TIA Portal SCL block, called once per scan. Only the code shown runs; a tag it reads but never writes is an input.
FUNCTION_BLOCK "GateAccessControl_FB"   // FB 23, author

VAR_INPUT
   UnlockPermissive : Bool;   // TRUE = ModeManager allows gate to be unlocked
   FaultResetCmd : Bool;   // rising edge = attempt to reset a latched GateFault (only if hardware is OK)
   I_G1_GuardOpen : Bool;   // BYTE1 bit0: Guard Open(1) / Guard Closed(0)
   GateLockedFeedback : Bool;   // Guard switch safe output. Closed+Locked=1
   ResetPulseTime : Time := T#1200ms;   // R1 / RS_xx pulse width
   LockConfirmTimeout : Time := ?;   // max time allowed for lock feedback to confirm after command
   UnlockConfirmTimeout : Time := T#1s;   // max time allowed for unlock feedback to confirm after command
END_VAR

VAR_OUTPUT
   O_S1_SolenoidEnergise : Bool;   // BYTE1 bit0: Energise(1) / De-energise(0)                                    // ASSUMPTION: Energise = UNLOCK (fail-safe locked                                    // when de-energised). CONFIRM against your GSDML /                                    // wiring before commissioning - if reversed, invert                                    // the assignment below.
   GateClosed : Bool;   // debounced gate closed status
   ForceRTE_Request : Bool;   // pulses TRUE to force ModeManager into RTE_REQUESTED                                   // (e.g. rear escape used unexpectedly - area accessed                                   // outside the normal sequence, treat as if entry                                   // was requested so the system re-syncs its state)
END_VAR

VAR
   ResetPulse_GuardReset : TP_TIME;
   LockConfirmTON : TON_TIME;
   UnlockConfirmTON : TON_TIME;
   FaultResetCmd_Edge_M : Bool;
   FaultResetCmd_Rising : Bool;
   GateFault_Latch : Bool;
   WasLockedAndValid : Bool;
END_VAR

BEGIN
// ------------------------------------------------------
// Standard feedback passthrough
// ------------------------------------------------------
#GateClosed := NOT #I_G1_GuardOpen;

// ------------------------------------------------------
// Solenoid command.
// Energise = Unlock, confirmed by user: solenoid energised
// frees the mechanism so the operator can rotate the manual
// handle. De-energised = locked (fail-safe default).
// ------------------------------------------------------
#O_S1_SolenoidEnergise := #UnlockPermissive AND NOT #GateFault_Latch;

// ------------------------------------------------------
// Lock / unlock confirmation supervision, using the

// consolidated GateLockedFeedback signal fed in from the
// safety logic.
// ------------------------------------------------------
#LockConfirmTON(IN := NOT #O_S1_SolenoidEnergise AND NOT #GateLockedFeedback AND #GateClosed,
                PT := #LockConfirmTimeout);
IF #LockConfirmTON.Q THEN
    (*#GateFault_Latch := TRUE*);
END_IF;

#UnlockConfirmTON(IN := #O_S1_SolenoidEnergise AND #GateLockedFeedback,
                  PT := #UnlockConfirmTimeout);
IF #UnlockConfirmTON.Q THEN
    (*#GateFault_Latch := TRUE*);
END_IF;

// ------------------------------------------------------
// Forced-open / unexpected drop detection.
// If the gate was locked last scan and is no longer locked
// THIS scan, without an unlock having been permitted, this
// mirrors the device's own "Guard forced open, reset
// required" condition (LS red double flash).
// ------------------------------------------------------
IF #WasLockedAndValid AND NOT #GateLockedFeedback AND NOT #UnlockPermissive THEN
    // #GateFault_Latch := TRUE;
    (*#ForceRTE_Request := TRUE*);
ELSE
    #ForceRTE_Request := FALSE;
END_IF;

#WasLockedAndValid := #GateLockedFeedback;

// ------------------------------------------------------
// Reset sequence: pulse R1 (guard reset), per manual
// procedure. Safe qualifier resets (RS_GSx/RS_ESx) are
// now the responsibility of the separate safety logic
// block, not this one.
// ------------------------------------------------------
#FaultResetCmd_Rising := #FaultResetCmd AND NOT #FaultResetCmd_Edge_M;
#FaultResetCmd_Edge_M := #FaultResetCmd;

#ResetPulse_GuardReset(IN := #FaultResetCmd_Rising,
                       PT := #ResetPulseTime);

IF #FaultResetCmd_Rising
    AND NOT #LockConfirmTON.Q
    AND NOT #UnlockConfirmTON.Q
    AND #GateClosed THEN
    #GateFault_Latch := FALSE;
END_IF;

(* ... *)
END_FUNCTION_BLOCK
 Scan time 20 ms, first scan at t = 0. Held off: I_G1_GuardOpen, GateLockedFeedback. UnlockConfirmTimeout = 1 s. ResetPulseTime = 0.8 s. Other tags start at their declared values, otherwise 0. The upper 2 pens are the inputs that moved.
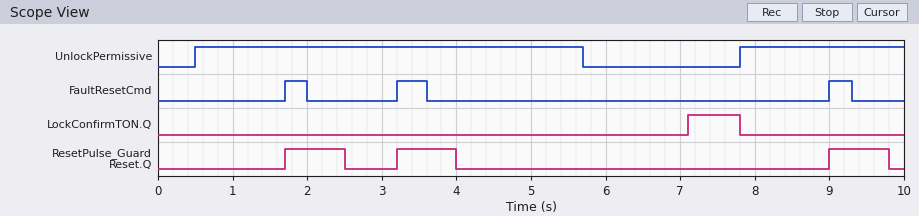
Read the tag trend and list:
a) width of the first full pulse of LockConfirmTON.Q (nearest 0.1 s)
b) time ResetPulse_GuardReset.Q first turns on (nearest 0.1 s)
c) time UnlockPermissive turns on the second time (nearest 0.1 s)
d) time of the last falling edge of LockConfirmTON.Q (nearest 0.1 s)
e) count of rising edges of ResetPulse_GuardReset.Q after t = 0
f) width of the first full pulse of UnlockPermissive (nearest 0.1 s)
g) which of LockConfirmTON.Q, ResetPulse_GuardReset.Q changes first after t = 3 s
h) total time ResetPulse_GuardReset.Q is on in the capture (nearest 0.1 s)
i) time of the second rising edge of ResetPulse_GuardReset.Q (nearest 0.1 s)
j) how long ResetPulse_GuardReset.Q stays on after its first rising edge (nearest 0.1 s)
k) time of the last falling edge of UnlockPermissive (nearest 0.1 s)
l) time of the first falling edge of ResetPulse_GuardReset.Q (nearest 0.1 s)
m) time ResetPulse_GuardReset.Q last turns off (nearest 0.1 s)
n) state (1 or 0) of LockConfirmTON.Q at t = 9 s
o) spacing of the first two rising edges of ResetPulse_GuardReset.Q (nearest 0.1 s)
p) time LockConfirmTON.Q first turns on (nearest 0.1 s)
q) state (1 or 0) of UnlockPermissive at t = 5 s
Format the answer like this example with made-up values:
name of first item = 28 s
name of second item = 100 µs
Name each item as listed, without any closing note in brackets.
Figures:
width of the first full pulse of LockConfirmTON.Q = 0.7 s
time ResetPulse_GuardReset.Q first turns on = 1.7 s
time UnlockPermissive turns on the second time = 7.8 s
time of the last falling edge of LockConfirmTON.Q = 7.8 s
count of rising edges of ResetPulse_GuardReset.Q after t = 0 = 3
width of the first full pulse of UnlockPermissive = 5.2 s
which of LockConfirmTON.Q, ResetPulse_GuardReset.Q changes first after t = 3 s = ResetPulse_GuardReset.Q
total time ResetPulse_GuardReset.Q is on in the capture = 2.4 s
time of the second rising edge of ResetPulse_GuardReset.Q = 3.2 s
how long ResetPulse_GuardReset.Q stays on after its first rising edge = 0.8 s
time of the last falling edge of UnlockPermissive = 5.7 s
time of the first falling edge of ResetPulse_GuardReset.Q = 2.5 s
time ResetPulse_GuardReset.Q last turns off = 9.8 s
state (1 or 0) of LockConfirmTON.Q at t = 9 s = 0
spacing of the first two rising edges of ResetPulse_GuardReset.Q = 1.5 s
time LockConfirmTON.Q first turns on = 7.1 s
state (1 or 0) of UnlockPermissive at t = 5 s = 1
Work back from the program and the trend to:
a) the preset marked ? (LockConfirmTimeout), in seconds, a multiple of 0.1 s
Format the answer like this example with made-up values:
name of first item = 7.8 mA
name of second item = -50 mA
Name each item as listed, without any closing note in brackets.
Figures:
the preset marked ? (LockConfirmTimeout), in seconds, a multiple of 0.1 s = 1.4 s
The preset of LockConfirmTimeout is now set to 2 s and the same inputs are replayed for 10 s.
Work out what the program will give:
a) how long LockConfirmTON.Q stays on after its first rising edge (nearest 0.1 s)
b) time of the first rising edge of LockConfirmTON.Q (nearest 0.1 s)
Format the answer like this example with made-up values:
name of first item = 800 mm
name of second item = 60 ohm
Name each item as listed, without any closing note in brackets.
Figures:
how long LockConfirmTON.Q stays on after its first rising edge = 0.1 s
time of the first rising edge of LockConfirmTON.Q = 7.7 s
